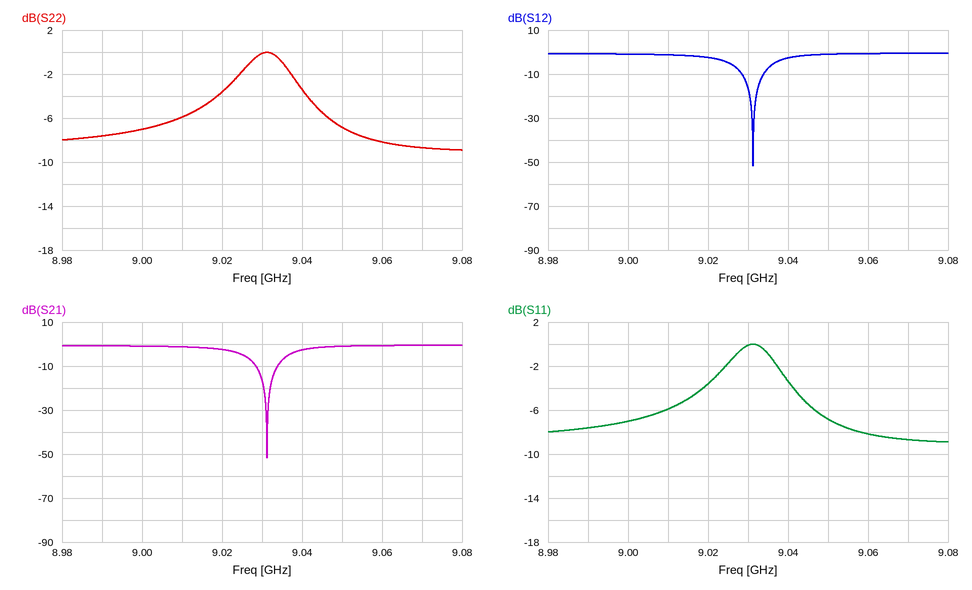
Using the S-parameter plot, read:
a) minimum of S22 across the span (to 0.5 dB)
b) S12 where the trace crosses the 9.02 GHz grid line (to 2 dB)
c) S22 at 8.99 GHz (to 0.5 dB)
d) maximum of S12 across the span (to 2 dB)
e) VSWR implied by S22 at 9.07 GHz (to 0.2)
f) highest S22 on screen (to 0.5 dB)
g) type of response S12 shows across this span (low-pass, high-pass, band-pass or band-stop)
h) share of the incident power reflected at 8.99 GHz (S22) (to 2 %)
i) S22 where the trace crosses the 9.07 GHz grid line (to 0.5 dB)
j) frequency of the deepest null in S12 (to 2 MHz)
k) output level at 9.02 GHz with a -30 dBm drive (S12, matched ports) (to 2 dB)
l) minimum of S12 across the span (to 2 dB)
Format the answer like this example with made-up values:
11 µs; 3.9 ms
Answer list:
-9.0 dB; -2 dB; -7.5 dB; 0 dB; 2.2; 0.0 dB; band-stop; 18 %; -8.5 dB; 9.032 GHz; -32 dBm; -52 dB
